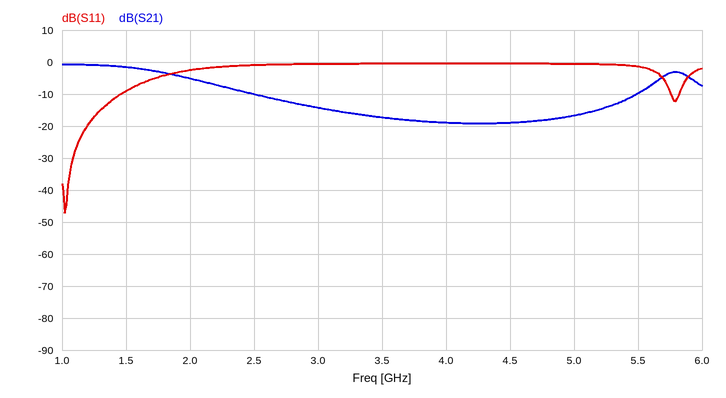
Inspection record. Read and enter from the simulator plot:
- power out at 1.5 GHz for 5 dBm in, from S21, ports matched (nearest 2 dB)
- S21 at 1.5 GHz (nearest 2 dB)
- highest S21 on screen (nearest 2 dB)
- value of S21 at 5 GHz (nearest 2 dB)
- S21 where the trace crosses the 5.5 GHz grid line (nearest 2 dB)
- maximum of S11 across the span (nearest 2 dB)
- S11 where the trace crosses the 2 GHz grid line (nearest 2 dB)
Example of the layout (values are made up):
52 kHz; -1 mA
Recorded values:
4 dBm; -2 dB; 0 dB; -16 dB; -10 dB; 0 dB; -2 dB
